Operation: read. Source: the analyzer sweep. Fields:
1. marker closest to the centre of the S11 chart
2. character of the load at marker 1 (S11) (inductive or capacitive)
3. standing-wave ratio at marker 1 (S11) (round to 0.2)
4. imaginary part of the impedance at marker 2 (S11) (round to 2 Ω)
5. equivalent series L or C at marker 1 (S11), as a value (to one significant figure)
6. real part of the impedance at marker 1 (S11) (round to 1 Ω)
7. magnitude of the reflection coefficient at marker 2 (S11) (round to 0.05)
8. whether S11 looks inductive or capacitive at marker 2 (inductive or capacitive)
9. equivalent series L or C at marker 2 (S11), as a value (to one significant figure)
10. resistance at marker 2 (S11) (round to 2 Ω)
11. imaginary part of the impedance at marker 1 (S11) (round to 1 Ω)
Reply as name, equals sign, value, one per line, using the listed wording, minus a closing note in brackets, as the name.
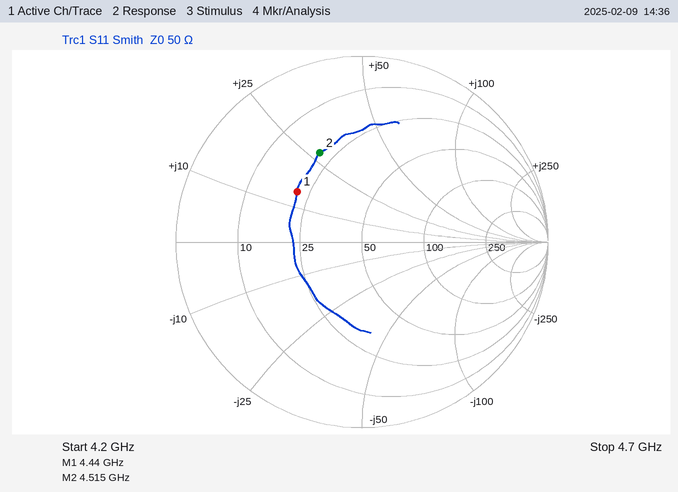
marker closest to the centre of the S11 chart = marker 1
character of the load at marker 1 (S11) = inductive
standing-wave ratio at marker 1 (S11) = 2.6
imaginary part of the impedance at marker 2 (S11) = +28 Ω
equivalent series L or C at marker 1 (S11), as a value = 500 pH
real part of the impedance at marker 1 (S11) = 21 Ω
magnitude of the reflection coefficient at marker 2 (S11) = 0.55
whether S11 looks inductive or capacitive at marker 2 = inductive
equivalent series L or C at marker 2 (S11), as a value = 1.0 nH
resistance at marker 2 (S11) = 20 Ω
imaginary part of the impedance at marker 1 (S11) = +14 Ω
